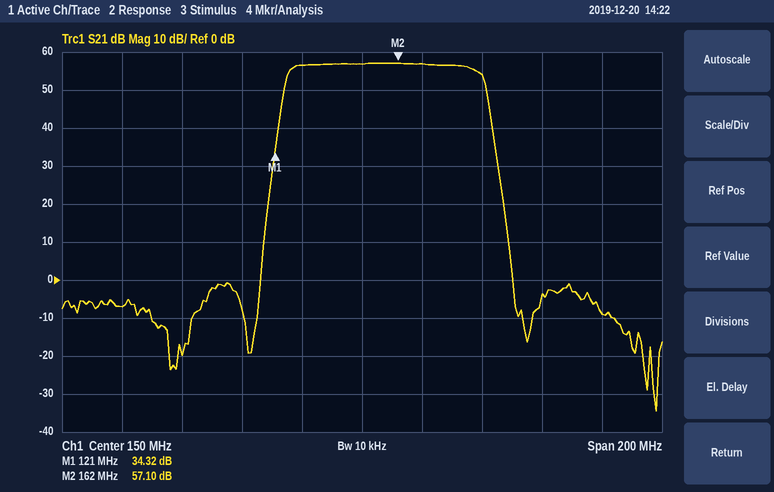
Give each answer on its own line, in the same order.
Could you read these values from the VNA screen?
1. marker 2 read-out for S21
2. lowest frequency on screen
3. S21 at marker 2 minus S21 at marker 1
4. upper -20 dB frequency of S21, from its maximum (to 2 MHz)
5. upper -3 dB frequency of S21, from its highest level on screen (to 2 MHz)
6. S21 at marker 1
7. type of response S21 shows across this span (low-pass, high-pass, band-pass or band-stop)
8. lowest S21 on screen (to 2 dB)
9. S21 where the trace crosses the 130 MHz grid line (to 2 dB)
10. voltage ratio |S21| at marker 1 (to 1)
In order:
57.10 dB
50 MHz
22.78 dB
194 MHz
190 MHz
34.32 dB
band-pass
-34 dB
56 dB
52
